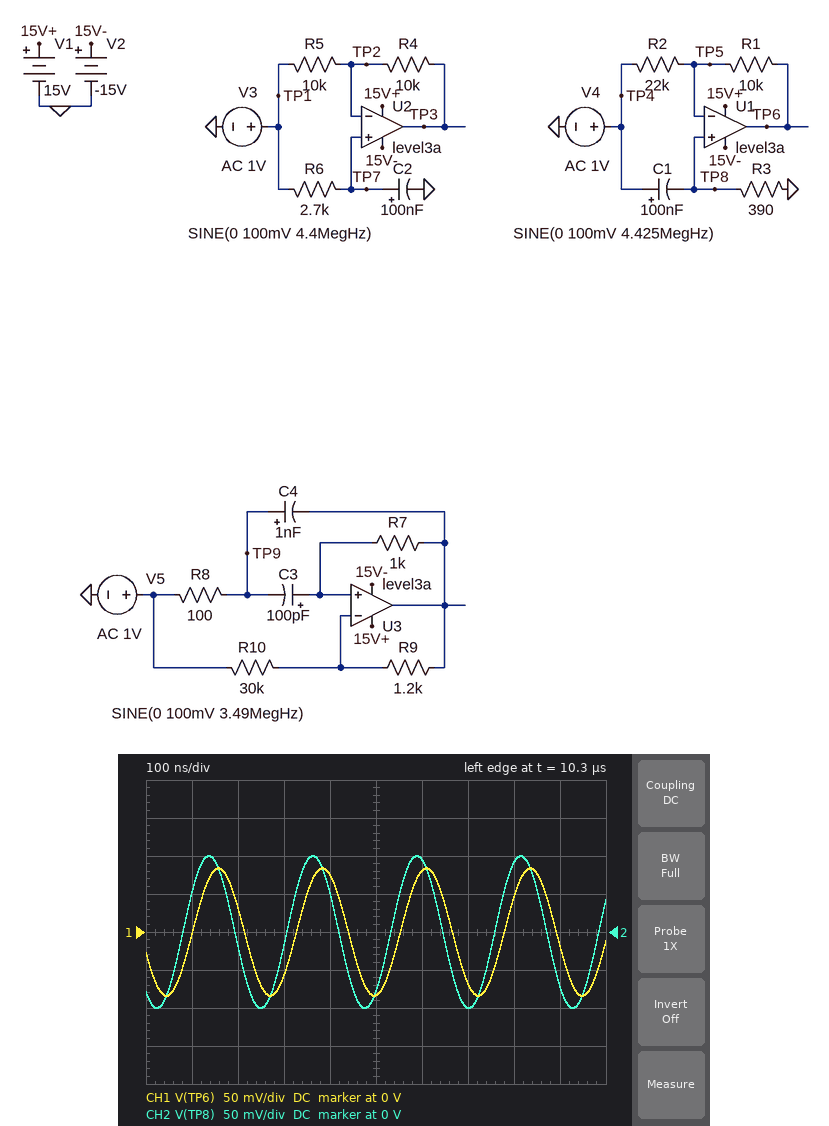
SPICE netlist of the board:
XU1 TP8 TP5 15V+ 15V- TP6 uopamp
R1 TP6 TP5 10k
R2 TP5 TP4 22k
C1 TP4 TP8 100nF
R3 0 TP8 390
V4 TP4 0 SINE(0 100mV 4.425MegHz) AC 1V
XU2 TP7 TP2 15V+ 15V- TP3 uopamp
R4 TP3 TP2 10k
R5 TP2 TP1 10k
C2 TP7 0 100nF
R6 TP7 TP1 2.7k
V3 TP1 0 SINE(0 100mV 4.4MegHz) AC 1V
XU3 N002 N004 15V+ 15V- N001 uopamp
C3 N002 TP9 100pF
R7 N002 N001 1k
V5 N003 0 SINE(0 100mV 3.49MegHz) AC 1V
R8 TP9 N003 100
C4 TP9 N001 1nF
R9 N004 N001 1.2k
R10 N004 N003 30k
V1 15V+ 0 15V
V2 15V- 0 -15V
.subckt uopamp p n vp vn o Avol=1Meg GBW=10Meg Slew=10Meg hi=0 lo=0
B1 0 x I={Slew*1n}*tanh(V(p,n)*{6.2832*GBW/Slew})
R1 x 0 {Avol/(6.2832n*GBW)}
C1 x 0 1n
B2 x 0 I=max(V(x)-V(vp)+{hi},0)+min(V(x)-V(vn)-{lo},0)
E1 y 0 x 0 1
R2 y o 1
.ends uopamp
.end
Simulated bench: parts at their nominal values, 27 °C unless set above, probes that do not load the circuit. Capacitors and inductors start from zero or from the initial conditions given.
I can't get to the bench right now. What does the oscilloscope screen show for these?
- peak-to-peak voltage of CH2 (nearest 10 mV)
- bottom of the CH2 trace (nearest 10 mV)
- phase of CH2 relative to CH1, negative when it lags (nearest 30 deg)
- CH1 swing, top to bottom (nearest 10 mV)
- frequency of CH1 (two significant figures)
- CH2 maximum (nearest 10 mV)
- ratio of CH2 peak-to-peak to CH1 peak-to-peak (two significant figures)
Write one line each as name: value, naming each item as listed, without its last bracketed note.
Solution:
peak-to-peak voltage of CH2: 200 mV
bottom of the CH2 trace: -100 mV
phase of CH2 relative to CH1, negative when it lags: 30 deg
CH1 swing, top to bottom: 170 mV
frequency of CH1: 4.4 MHz
CH2 maximum: 100 mV
ratio of CH2 peak-to-peak to CH1 peak-to-peak: 1.2
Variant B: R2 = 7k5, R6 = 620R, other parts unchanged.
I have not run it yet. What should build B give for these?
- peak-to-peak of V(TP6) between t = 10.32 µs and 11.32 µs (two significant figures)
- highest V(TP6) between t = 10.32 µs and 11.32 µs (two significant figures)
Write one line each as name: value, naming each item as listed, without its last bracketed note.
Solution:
peak-to-peak of V(TP6) between t = 10.32 µs and 11.32 µs: 140 mV
highest V(TP6) between t = 10.32 µs and 11.32 µs: 69 mV
